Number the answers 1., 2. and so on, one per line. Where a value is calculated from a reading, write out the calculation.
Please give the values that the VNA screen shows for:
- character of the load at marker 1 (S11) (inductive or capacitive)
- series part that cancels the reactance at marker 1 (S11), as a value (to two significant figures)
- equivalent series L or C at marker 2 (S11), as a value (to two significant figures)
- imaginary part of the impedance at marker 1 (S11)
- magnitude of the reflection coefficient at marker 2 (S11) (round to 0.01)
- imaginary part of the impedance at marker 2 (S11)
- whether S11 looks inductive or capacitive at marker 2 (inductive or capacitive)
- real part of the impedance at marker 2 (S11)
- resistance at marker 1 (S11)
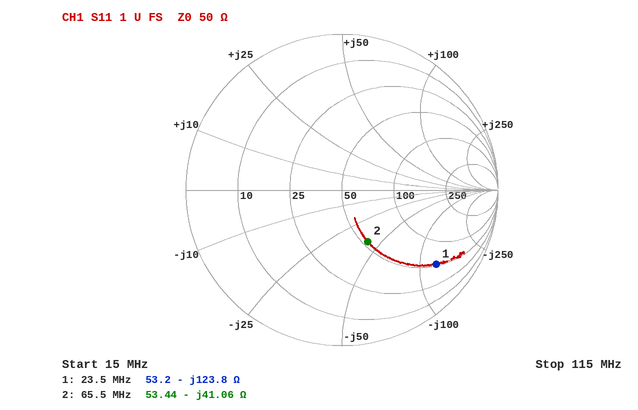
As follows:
1. capacitive
2. L = 123.8 Ω/(2π × 23.5 MHz) ≈ 838 nH, so 840 nH to two significant figures
3. C = 1/(2π × 65.5 MHz × 41.06 Ω) ≈ 59 pF
4. -123.8 Ω
5. 0.37
6. -41.06 Ω
7. capacitive
8. 53.44 Ω
9. 53.2 Ω
